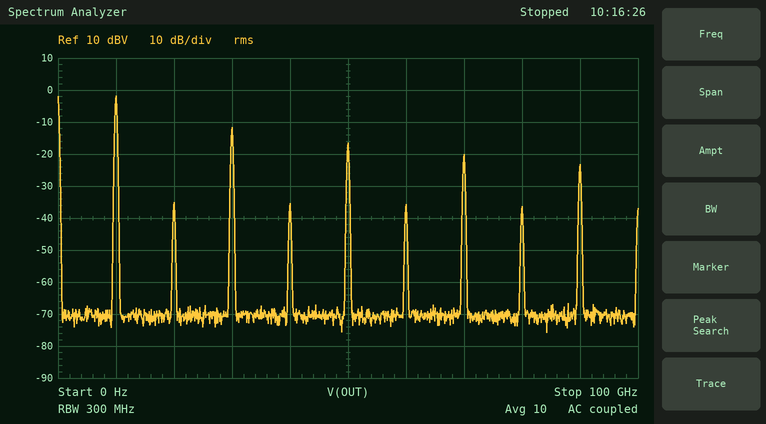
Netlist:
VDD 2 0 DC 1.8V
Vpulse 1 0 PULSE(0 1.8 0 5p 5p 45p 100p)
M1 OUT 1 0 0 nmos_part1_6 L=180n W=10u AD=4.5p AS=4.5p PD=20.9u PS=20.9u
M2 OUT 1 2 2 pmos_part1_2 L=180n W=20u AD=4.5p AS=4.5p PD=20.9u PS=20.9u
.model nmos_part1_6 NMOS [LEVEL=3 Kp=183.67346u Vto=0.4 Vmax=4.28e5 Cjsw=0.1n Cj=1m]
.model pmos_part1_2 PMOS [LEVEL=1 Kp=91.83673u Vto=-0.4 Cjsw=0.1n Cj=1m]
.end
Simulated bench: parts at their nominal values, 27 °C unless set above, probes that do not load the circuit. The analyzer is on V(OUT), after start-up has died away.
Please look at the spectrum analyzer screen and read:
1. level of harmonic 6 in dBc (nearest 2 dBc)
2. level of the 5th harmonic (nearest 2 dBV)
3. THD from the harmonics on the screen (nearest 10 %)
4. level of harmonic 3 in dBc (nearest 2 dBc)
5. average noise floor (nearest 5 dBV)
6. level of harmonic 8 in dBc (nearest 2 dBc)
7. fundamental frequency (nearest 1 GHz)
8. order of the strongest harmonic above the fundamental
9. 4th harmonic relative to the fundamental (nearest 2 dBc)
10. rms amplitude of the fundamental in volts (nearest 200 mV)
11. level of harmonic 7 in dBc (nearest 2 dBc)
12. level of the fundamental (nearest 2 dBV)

-34 dBc
-16 dBV
40 %
-10 dBc
-70 dBV
-34 dBc
10 GHz
3
-34 dBc
800 mV
-18 dBc
-2 dBV
